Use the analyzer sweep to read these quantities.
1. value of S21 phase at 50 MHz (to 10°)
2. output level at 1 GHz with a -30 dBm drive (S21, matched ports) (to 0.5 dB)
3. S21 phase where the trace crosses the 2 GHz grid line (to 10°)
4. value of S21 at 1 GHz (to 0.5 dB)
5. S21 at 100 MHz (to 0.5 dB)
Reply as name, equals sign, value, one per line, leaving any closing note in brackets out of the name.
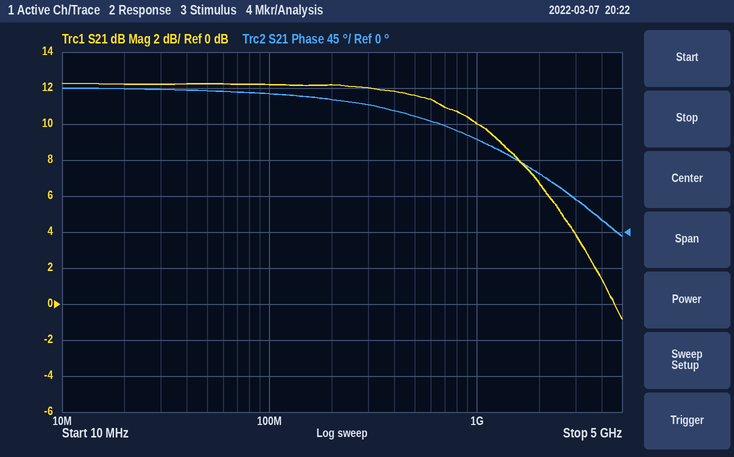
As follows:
value of S21 phase at 50 MHz = 180°
output level at 1 GHz with a -30 dBm drive (S21, matched ports) = -20.0 dBm
S21 phase where the trace crosses the 2 GHz grid line = 70°
value of S21 at 1 GHz = 10.0 dB
S21 at 100 MHz = 12.0 dB
